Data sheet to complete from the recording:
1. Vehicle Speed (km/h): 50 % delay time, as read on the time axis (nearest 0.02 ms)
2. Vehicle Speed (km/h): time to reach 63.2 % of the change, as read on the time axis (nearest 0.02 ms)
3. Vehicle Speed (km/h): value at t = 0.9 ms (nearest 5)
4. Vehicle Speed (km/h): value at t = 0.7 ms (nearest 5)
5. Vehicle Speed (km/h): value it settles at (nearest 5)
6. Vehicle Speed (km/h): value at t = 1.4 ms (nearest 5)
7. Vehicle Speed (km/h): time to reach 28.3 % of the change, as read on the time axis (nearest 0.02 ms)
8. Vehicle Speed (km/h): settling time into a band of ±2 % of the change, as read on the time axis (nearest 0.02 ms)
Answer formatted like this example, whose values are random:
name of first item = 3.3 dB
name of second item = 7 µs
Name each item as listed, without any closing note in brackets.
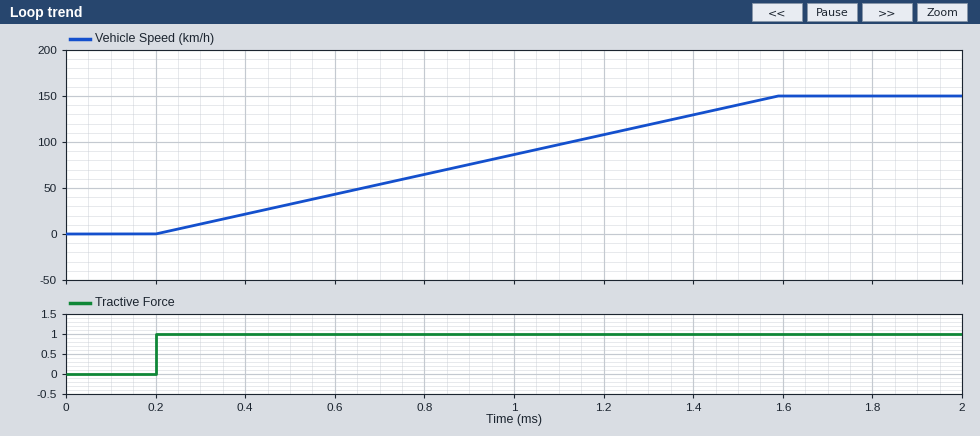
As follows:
Vehicle Speed (km/h): 50 % delay time, as read on the time axis = 0.90 ms
Vehicle Speed (km/h): time to reach 63.2 % of the change, as read on the time axis = 1.08 ms
Vehicle Speed (km/h): value at t = 0.9 ms = 75
Vehicle Speed (km/h): value at t = 0.7 ms = 55
Vehicle Speed (km/h): value it settles at = 150
Vehicle Speed (km/h): value at t = 1.4 ms = 130
Vehicle Speed (km/h): time to reach 28.3 % of the change, as read on the time axis = 0.60 ms
Vehicle Speed (km/h): settling time into a band of ±2 % of the change, as read on the time axis = 1.56 ms
